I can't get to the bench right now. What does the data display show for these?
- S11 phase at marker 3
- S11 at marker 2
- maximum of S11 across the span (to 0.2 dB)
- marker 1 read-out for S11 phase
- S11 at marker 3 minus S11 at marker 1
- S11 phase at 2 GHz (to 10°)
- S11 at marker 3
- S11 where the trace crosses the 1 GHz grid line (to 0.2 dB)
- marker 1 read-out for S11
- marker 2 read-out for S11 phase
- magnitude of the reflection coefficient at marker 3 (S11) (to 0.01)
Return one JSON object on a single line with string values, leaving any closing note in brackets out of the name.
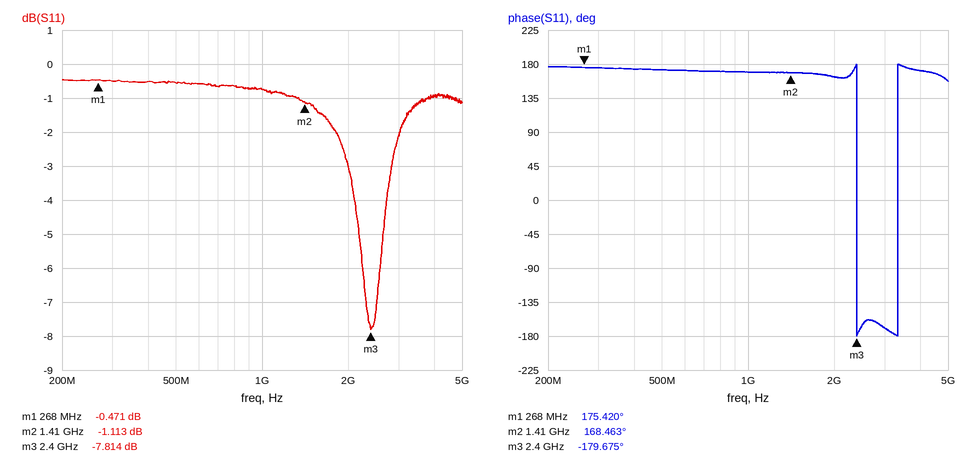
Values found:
{"S11 phase at marker 3": "-179.675°", "S11 at marker 2": "-1.113 dB", "maximum of S11 across the span": "-0.4 dB", "marker 1 read-out for S11 phase": "175.420°", "S11 at marker 3 minus S11 at marker 1": "-7.343 dB", "S11 phase at 2 GHz": "160°", "S11 at marker 3": "-7.814 dB", "S11 where the trace crosses the 1 GHz grid line": "-0.8 dB", "marker 1 read-out for S11": "-0.471 dB", "marker 2 read-out for S11 phase": "168.463°", "magnitude of the reflection coefficient at marker 3 (S11)": "0.41"}
